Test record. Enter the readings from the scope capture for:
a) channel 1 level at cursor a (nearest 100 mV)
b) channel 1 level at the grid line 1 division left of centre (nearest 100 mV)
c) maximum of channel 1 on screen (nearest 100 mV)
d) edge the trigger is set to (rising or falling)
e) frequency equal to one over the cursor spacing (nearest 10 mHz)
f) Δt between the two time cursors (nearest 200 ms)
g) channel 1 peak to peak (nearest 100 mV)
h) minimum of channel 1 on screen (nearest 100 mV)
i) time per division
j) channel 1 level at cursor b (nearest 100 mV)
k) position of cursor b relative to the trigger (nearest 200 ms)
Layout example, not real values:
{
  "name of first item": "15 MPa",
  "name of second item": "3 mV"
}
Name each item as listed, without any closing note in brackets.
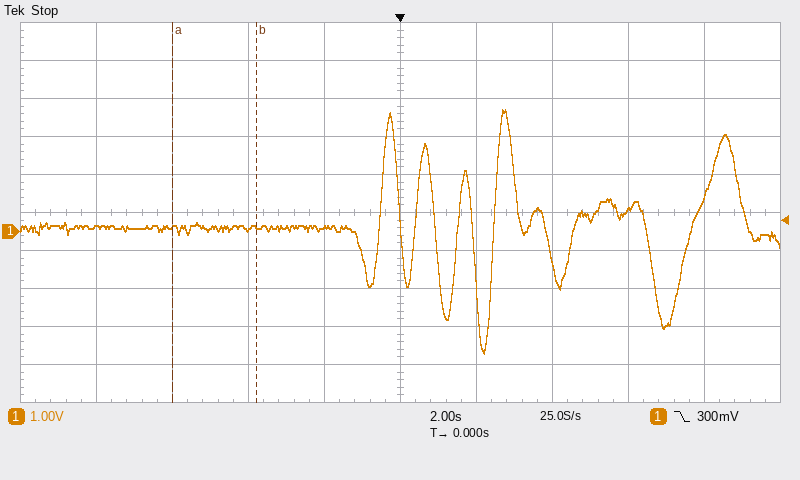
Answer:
{
  "channel 1 level at cursor a": "100 mV",
  "channel 1 level at the grid line 1 division left of centre": "100 mV",
  "maximum of channel 1 on screen": "3.2 V",
  "edge the trigger is set to": "falling",
  "frequency equal to one over the cursor spacing": "450 mHz",
  "Δt between the two time cursors": "2.2 s",
  "channel 1 peak to peak": "6.4 V",
  "minimum of channel 1 on screen": "-3.2 V",
  "time per division": "2 s",
  "channel 1 level at cursor b": "100 mV",
  "position of cursor b relative to the trigger": "-3.8 s"
}
